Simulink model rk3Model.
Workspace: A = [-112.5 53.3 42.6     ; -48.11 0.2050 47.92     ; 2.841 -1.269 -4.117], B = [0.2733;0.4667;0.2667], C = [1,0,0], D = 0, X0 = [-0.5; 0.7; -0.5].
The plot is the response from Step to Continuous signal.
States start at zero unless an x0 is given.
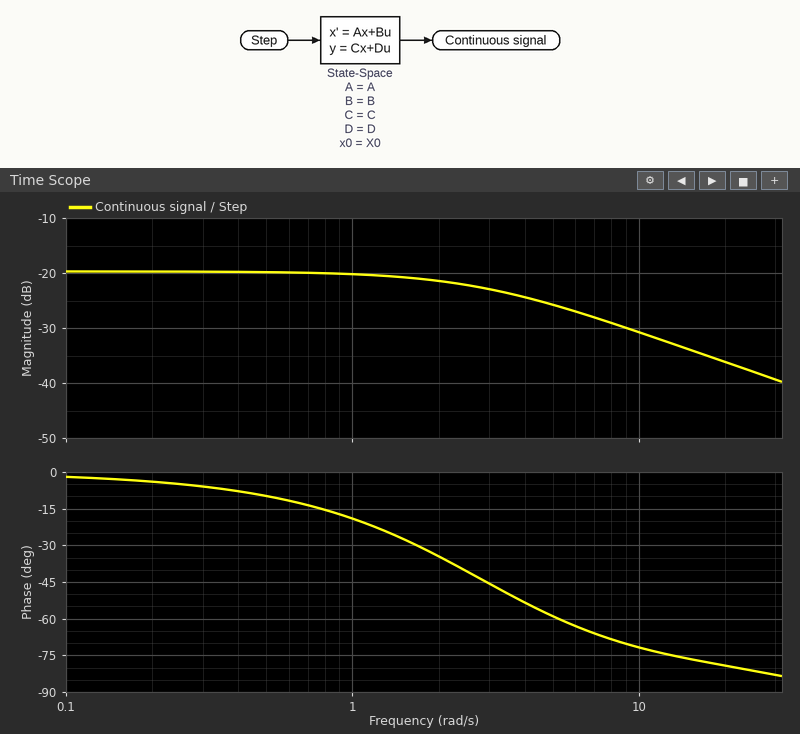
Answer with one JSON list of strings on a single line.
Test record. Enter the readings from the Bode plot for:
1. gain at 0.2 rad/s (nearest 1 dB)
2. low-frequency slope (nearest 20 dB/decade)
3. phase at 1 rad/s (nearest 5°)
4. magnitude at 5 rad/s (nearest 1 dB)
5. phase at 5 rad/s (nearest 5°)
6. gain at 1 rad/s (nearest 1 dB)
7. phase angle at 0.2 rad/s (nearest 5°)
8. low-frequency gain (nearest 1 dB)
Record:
["-20 dB", "0 dB/decade", "-20°", "-26 dB", "-60°", "-20 dB", "-5°", "-20 dB"]
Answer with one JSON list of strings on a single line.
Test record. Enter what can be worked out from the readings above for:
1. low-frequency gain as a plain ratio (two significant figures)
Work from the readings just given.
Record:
["0.10"]
